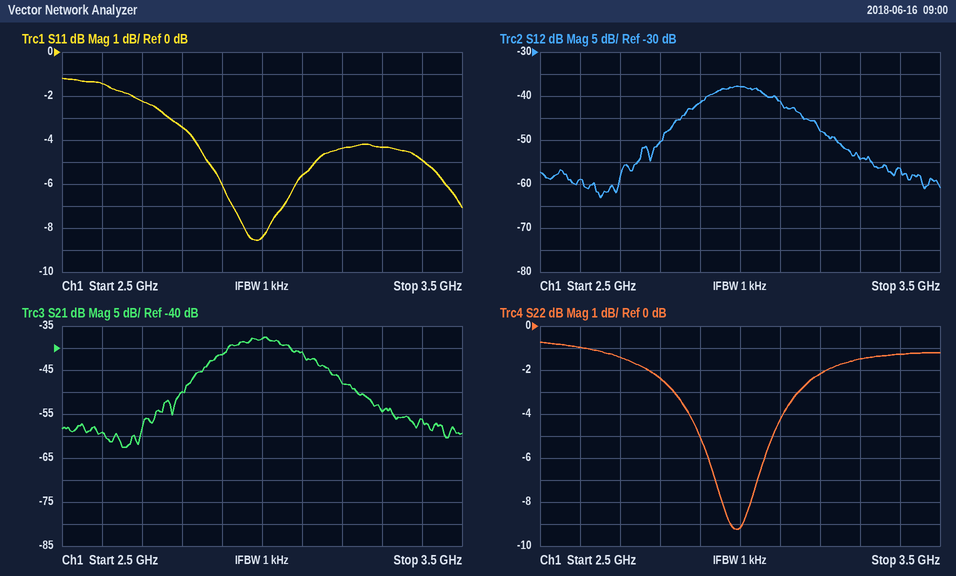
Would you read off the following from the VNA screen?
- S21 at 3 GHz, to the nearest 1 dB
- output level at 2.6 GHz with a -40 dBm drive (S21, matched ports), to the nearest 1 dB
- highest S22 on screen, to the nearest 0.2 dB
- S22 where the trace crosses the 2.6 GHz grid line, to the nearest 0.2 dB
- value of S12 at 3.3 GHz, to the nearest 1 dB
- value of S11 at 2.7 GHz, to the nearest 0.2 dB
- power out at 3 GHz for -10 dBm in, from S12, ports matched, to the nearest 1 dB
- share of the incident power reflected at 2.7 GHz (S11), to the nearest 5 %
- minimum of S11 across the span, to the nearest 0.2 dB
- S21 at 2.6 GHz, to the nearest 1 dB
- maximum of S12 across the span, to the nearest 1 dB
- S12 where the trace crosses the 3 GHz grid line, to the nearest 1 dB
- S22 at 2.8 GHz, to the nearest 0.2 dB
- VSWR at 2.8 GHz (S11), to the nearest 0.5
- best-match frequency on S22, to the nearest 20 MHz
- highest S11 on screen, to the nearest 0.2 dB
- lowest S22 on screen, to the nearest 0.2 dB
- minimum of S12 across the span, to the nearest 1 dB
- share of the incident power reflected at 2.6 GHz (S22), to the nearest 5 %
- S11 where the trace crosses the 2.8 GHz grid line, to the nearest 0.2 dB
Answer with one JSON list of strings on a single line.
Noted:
["-38 dB", "-99 dBm", "-0.8 dB", "-1.0 dB", "-54 dB", "-2.2 dB", "-48 dBm", "60 %", "-8.6 dB", "-59 dB", "-38 dB", "-38 dB", "-2.4 dB", "5.0", "3.00 GHz", "-1.2 dB", "-9.2 dB", "-63 dB", "80 %", "-3.4 dB"]
